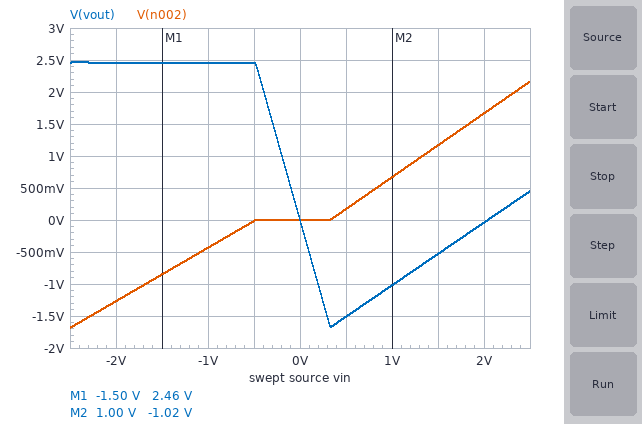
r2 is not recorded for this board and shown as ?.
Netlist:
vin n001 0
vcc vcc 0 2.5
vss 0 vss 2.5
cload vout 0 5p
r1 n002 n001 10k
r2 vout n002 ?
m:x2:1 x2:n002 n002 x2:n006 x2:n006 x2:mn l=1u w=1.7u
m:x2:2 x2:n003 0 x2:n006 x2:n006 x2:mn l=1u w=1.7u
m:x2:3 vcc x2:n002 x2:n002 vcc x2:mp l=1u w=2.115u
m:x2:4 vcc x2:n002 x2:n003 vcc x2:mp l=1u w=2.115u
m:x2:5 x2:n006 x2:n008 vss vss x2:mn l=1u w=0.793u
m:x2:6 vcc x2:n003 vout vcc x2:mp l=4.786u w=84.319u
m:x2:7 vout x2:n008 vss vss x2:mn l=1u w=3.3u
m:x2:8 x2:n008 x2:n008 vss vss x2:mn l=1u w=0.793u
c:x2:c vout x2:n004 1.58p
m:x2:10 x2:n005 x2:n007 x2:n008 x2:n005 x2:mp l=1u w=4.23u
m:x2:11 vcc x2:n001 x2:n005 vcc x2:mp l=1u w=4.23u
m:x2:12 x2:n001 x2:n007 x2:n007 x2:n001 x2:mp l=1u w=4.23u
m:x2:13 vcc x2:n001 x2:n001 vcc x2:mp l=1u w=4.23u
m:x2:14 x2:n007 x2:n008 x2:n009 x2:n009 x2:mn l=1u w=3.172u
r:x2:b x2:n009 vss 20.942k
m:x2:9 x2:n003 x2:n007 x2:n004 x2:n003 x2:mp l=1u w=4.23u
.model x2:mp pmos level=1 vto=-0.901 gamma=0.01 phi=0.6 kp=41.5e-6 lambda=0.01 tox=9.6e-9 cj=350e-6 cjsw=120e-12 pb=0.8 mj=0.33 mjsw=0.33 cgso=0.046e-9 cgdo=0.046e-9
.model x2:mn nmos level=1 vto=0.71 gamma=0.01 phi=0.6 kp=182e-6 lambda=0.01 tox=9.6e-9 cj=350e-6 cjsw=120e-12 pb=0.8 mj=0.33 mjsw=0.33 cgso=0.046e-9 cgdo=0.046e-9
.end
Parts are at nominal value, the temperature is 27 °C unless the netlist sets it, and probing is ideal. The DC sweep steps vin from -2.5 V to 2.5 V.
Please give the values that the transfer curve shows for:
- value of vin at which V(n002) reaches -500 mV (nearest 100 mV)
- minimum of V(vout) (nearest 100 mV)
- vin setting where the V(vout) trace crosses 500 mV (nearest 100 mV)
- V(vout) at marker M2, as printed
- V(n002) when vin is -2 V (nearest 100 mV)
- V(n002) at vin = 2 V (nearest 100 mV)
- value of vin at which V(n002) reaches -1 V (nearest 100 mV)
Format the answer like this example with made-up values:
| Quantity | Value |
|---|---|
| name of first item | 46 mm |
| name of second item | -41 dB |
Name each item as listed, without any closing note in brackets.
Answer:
| Quantity | Value |
|---|---|
| value of vin at which V(n002) reaches -500 mV | -1.1 V |
| minimum of V(vout) | -1.7 V |
| vin setting where the V(vout) trace crosses 500 mV | -100 mV |
| V(vout) at marker M2, as printed | -1.02 V |
| V(n002) when vin is -2 V | -1.3 V |
| V(n002) at vin = 2 V | 1.7 V |
| value of vin at which V(n002) reaches -1 V | -1.7 V |
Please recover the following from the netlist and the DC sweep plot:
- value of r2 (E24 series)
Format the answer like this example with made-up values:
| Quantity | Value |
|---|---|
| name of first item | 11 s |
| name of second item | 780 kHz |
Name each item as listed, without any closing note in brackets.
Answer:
| Quantity | Value |
|---|---|
| value of r2 | 51 kΩ |
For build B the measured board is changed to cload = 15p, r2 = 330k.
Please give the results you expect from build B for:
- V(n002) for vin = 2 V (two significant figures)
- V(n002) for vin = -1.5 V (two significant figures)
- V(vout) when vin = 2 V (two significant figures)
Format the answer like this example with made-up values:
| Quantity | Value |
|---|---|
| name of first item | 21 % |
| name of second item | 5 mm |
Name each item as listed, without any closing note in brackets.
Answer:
| Quantity | Value |
|---|---|
| V(n002) for vin = 2 V | 1.9 V |
| V(n002) for vin = -1.5 V | -1.4 V |
| V(vout) when vin = 2 V | -2.4 V |
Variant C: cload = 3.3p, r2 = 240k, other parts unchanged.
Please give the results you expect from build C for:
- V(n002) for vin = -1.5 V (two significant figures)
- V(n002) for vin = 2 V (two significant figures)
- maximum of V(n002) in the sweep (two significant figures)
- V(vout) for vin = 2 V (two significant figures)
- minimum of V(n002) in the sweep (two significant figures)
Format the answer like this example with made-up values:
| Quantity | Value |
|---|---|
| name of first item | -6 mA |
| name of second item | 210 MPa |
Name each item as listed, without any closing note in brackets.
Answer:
| Quantity | Value |
|---|---|
| V(n002) for vin = -1.5 V | -1.3 V |
| V(n002) for vin = 2 V | 1.8 V |
| maximum of V(n002) in the sweep | 2.3 V |
| V(vout) for vin = 2 V | -2.4 V |
| minimum of V(n002) in the sweep | -2.3 V |
